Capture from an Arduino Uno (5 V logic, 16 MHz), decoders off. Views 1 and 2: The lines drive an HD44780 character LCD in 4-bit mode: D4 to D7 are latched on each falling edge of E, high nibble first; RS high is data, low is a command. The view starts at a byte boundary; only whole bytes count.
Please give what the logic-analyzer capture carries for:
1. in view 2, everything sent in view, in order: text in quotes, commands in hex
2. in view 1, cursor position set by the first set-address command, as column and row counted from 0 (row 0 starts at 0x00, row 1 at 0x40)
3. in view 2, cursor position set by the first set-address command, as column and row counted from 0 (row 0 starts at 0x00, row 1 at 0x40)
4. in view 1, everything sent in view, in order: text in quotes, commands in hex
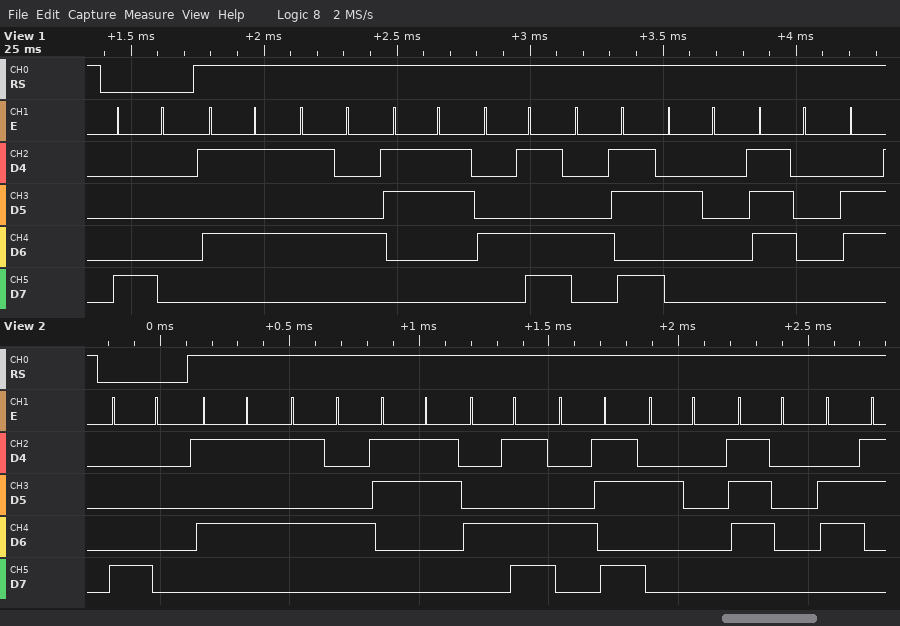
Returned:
0x80 "UT3MK pc"
column 0, row 0
column 0, row 0
0x80 "UT3MK p"
